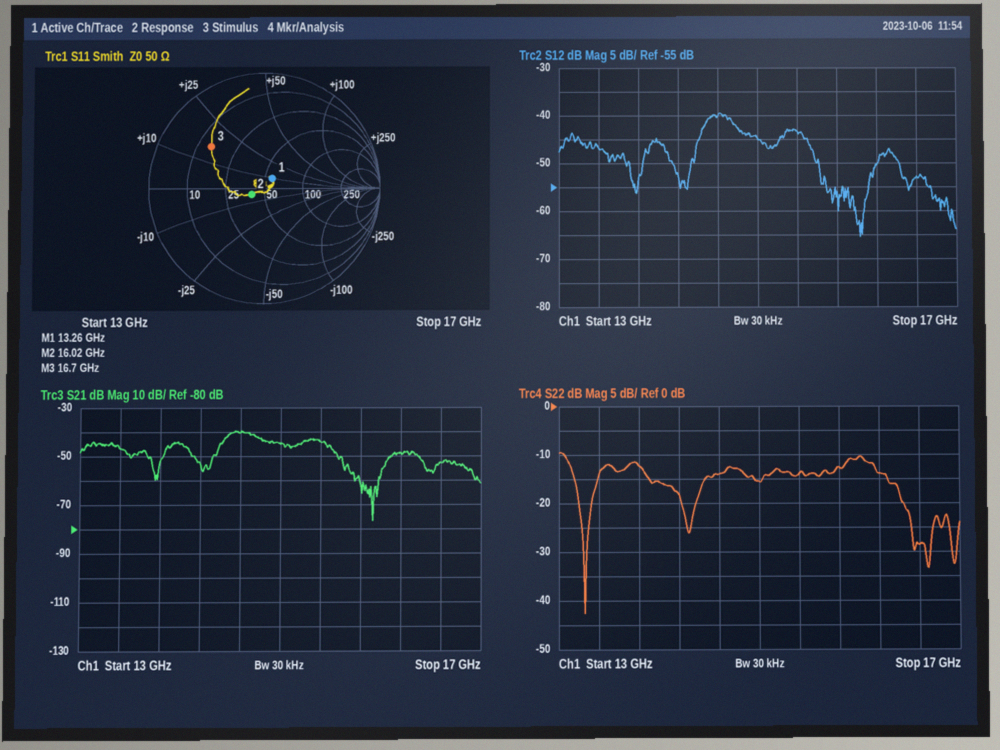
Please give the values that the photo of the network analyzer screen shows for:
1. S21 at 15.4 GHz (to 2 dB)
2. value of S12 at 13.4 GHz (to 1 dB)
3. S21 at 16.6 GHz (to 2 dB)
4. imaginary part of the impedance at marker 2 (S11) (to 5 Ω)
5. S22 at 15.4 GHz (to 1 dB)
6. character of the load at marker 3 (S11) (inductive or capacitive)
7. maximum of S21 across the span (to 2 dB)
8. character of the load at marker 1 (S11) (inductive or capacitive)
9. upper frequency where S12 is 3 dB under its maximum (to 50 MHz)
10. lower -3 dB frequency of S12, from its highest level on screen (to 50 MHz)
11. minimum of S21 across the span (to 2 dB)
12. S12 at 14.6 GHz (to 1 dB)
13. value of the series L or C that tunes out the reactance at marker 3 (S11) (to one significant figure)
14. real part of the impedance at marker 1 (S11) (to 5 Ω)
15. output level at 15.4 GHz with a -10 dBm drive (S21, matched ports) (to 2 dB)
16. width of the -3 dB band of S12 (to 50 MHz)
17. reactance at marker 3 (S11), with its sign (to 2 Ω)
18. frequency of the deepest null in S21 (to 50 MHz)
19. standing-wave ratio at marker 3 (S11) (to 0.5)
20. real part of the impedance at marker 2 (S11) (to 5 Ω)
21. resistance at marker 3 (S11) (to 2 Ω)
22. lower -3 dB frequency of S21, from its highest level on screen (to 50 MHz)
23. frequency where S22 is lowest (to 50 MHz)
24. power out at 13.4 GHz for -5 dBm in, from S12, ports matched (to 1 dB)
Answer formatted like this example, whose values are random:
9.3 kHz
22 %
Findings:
-44 dB
-47 dB
-52 dB
-5 Ω
-14 dB
inductive
-40 dB
inductive
14.80 GHz
14.45 GHz
-76 dB
-40 dB
600 fF
55 Ω
-54 dBm
350 MHz
+16 Ω
15.90 GHz
4.0
40 Ω
14 Ω
14.45 GHz
13.25 GHz
-52 dBm
